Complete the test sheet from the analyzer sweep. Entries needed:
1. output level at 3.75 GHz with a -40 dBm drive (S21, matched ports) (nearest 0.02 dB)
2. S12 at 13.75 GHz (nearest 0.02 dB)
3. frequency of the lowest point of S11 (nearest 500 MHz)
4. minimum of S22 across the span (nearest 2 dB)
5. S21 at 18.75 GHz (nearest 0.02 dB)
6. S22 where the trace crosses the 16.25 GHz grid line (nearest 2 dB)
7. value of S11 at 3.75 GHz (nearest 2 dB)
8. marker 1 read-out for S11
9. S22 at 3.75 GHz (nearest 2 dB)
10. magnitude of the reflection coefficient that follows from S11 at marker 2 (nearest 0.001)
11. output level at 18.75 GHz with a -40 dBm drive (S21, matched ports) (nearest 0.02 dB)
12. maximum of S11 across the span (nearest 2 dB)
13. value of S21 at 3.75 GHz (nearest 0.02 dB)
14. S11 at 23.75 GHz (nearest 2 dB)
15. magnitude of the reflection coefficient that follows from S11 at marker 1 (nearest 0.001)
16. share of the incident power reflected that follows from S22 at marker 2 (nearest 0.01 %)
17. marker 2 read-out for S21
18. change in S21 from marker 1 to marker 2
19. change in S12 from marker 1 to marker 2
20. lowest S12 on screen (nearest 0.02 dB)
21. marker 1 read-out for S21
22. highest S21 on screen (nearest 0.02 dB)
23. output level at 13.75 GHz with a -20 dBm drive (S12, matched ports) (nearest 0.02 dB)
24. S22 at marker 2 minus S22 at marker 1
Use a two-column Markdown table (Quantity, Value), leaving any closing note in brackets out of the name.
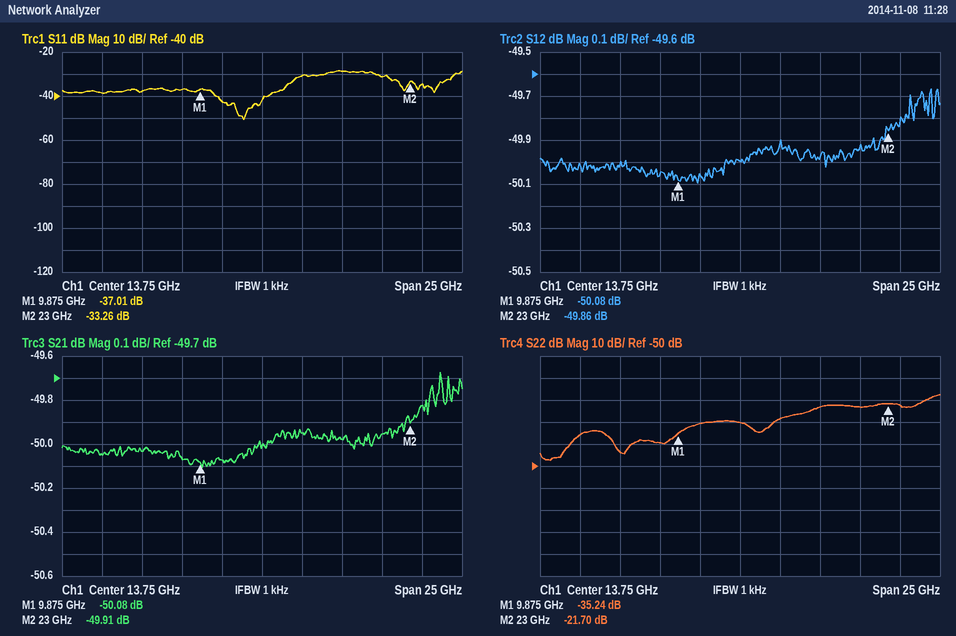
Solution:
| Quantity | Value |
|---|---|
| output level at 3.75 GHz with a -40 dBm drive (S21, matched ports) | -90.04 dBm |
| S12 at 13.75 GHz | -50.00 dB |
| frequency of the lowest point of S11 | 12.5 GHz |
| minimum of S22 across the span | -48 dB |
| S21 at 18.75 GHz | -49.98 dB |
| S22 where the trace crosses the 16.25 GHz grid line | -28 dB |
| value of S11 at 3.75 GHz | -38 dB |
| marker 1 read-out for S11 | -37.01 dB |
| S22 at 3.75 GHz | -36 dB |
| magnitude of the reflection coefficient that follows from S11 at marker 2 | 0.022 |
| output level at 18.75 GHz with a -40 dBm drive (S21, matched ports) | -89.98 dBm |
| maximum of S11 across the span | -28 dB |
| value of S21 at 3.75 GHz | -50.04 dB |
| S11 at 23.75 GHz | -34 dB |
| magnitude of the reflection coefficient that follows from S11 at marker 1 | 0.014 |
| share of the incident power reflected that follows from S22 at marker 2 | 0.68 % |
| marker 2 read-out for S21 | -49.91 dB |
| change in S21 from marker 1 to marker 2 | 0.17 dB |
| change in S12 from marker 1 to marker 2 | 0.22 dB |
| lowest S12 on screen | -50.10 dB |
| marker 1 read-out for S21 | -50.08 dB |
| highest S21 on screen | -49.68 dB |
| output level at 13.75 GHz with a -20 dBm drive (S12, matched ports) | -70.00 dBm |
| S22 at marker 2 minus S22 at marker 1 | 13.54 dB |
